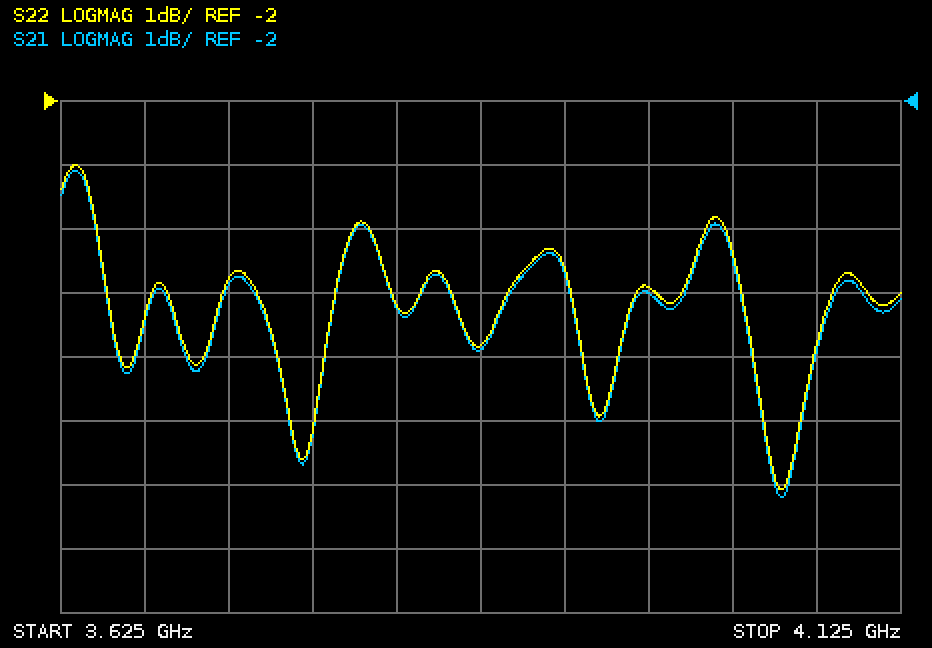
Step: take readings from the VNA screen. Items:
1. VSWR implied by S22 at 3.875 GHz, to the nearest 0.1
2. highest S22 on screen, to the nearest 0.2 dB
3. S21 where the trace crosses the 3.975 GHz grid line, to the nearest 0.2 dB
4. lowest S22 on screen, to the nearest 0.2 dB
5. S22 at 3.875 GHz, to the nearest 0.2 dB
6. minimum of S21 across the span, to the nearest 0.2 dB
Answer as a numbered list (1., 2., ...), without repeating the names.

1. 3.1
2. -3.0 dB
3. -5.0 dB
4. -8.0 dB
5. -5.8 dB
6. -8.2 dB
